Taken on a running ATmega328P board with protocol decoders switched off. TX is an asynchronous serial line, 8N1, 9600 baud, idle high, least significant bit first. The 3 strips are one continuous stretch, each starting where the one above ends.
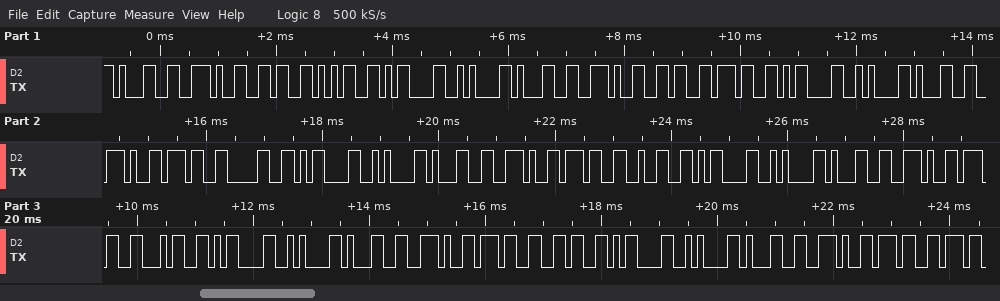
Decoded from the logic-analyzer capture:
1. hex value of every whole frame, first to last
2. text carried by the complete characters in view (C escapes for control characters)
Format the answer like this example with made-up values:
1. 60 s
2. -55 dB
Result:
1. 0x31 0x2E 0x36 0x35 0x0D 0x0A 0x31 0x2E 0x36 0x37 0x0D 0x0A 0x31 0x2E 0x37 0x30 0x0D 0x0A 0x31 0x2E 0x37 0x32 0x0D 0x0A 0x31 0x2E 0x37 0x34 0x0D 0x0A 0x31 0x2E 0x37 0x36 0x0D 0x0A 0x31 0x2E 0x37
2. "1.65\r\n1.67\r\n1.70\r\n1.72\r\n1.74\r\n1.76\r\n1.7"
